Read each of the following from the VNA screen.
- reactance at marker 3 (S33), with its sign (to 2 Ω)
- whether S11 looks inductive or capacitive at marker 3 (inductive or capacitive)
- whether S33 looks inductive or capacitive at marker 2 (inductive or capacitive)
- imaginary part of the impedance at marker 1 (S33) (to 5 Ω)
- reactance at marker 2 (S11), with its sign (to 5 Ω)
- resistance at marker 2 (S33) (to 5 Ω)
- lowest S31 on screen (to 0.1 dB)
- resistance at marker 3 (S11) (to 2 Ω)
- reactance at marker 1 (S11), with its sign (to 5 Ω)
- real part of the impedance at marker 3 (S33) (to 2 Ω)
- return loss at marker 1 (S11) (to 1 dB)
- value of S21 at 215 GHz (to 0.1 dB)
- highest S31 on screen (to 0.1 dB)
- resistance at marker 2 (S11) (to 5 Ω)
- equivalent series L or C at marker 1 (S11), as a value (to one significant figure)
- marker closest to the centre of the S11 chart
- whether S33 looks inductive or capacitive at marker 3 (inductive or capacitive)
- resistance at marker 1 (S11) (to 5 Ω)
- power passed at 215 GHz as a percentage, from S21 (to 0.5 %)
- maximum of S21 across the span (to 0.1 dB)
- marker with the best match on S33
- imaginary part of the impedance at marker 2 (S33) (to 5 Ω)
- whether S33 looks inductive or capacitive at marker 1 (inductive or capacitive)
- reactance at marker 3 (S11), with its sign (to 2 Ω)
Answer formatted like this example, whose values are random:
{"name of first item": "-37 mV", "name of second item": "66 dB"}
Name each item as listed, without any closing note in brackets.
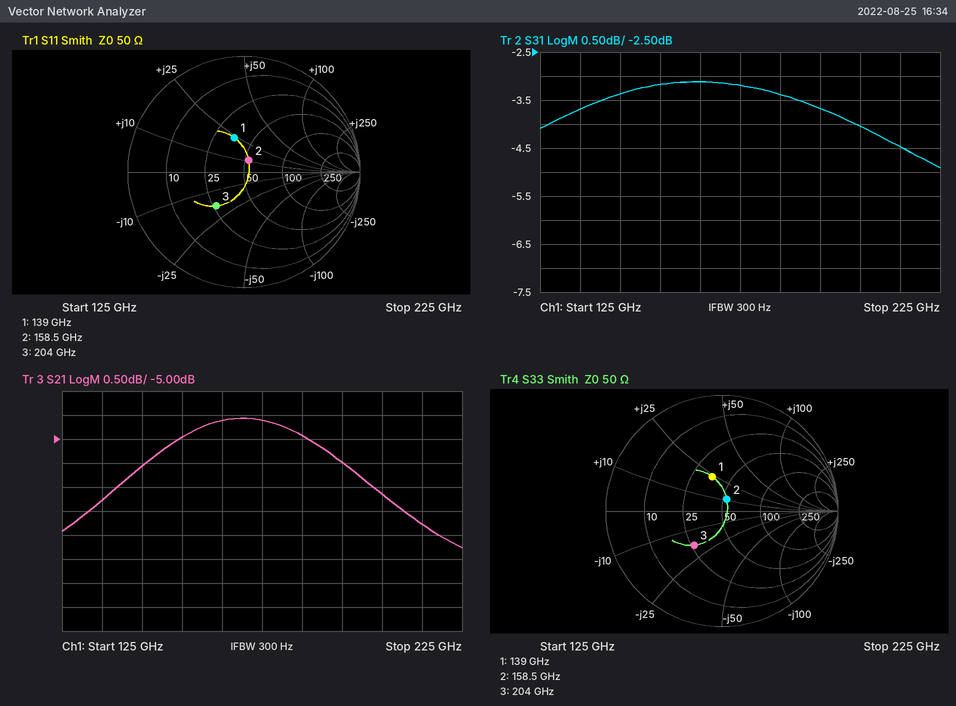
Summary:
{"reactance at marker 3 (S33), with its sign": "-18 Ω", "whether S11 looks inductive or capacitive at marker 3": "capacitive", "whether S33 looks inductive or capacitive at marker 2": "inductive", "imaginary part of the impedance at marker 1 (S33)": "+25 Ω", "reactance at marker 2 (S11), with its sign": "+10 Ω", "resistance at marker 2 (S33)": "55 Ω", "lowest S31 on screen": "-4.9 dB", "resistance at marker 3 (S11)": "26 Ω", "reactance at marker 1 (S11), with its sign": "+25 Ω", "real part of the impedance at marker 3 (S33)": "26 Ω", "return loss at marker 1 (S11)": "10 dB", "value of S21 at 215 GHz": "-6.8 dB", "highest S31 on screen": "-3.1 dB", "resistance at marker 2 (S11)": "55 Ω", "equivalent series L or C at marker 1 (S11), as a value": "30 pH", "marker closest to the centre of the S11 chart": "marker 2", "whether S33 looks inductive or capacitive at marker 3": "capacitive", "resistance at marker 1 (S11)": "35 Ω", "power passed at 215 GHz as a percentage, from S21": "21.0 %", "maximum of S21 across the span": "-4.6 dB", "marker with the best match on S33": "marker 2", "imaginary part of the impedance at marker 2 (S33)": "+10 Ω", "whether S33 looks inductive or capacitive at marker 1": "inductive", "reactance at marker 3 (S11), with its sign": "-18 Ω"}
